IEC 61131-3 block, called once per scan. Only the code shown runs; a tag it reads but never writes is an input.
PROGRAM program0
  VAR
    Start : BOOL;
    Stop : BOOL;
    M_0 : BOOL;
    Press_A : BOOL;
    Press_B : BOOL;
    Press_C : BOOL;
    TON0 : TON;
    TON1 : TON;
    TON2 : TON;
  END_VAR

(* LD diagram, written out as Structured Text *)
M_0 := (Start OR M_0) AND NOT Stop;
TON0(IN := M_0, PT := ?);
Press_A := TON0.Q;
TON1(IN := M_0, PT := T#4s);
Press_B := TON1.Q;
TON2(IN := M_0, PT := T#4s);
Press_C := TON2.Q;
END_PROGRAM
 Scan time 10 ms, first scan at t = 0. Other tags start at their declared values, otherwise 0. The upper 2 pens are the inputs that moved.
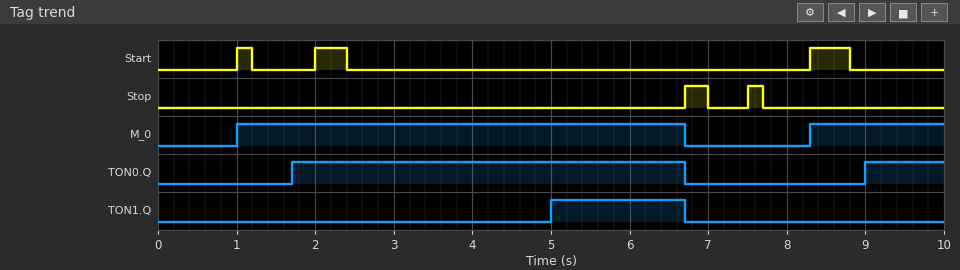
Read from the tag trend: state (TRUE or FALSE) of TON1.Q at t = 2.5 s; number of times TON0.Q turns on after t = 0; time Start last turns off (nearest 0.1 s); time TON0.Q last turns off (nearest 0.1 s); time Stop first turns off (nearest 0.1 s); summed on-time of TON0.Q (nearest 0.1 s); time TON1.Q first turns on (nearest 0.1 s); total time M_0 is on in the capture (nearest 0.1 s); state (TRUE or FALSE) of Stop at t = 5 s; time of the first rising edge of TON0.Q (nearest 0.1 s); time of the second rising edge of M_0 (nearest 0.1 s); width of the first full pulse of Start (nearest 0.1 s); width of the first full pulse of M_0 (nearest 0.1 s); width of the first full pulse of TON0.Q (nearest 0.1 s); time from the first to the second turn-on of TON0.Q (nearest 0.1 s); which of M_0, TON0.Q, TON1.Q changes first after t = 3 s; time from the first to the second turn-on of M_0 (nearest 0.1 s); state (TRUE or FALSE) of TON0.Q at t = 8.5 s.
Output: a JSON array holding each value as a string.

["FALSE", "2", "8.8 s", "6.7 s", "7.0 s", "6.0 s", "5.0 s", "7.4 s", "FALSE", "1.7 s", "8.3 s", "0.2 s", "5.7 s", "5.0 s", "7.3 s", "TON1.Q", "7.3 s", "FALSE"]
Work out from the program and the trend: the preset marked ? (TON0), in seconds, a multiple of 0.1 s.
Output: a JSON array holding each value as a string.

["0.7 s"]
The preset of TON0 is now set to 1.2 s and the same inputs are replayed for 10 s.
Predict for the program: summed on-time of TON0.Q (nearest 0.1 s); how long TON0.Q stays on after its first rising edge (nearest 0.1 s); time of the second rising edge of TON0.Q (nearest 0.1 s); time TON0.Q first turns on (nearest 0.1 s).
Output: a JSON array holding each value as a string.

["5.0 s", "4.5 s", "9.5 s", "2.2 s"]
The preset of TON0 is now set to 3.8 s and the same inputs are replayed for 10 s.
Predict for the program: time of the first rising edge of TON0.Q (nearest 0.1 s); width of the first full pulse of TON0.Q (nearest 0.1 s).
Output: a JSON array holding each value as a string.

["4.8 s", "1.9 s"]
